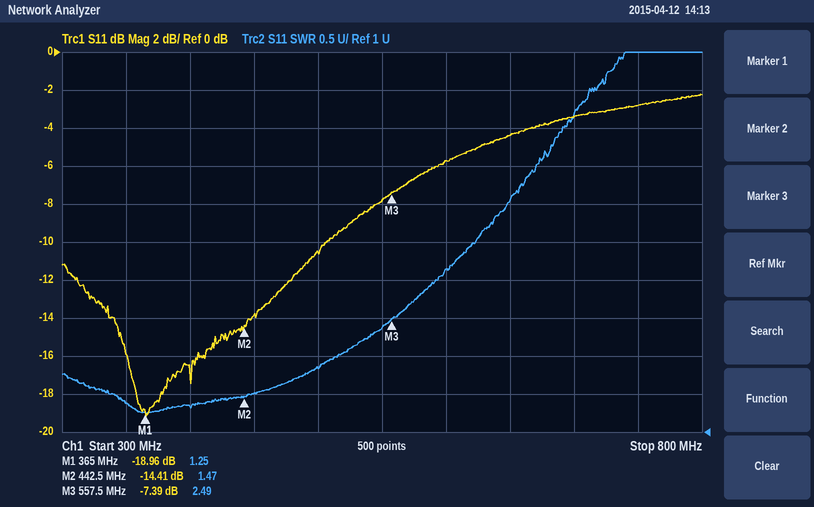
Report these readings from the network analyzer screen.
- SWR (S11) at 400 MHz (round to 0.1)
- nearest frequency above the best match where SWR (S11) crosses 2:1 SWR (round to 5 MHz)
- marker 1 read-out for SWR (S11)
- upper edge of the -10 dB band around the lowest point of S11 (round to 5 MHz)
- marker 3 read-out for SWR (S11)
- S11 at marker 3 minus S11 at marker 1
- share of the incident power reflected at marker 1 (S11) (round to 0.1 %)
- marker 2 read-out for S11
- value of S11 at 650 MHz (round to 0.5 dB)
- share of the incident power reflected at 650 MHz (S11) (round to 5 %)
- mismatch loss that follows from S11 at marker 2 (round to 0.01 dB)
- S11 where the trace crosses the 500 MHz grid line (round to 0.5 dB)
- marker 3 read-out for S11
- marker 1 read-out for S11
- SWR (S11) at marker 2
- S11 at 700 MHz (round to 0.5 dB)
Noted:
1.3
515 MHz
1.25
505 MHz
2.49
11.57 dB
1.3 %
-14.41 dB
-4.5 dB
35 %
0.16 dB
-10.5 dB
-7.39 dB
-18.96 dB
1.47
-3.5 dB
